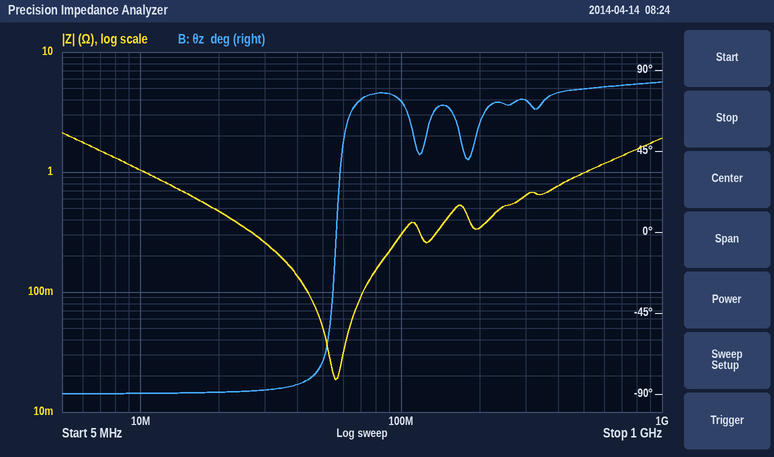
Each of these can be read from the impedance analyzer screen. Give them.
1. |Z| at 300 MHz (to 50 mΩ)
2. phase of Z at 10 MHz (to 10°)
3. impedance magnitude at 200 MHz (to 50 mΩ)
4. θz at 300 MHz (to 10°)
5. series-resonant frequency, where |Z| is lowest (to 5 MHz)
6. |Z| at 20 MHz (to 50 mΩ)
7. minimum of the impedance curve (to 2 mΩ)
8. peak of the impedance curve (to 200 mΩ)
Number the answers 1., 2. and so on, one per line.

1. 650 mΩ
2. -90°
3. 350 mΩ
4. 70°
5. 55 MHz
6. 450 mΩ
7. 18 mΩ
8. 2.2 Ω
